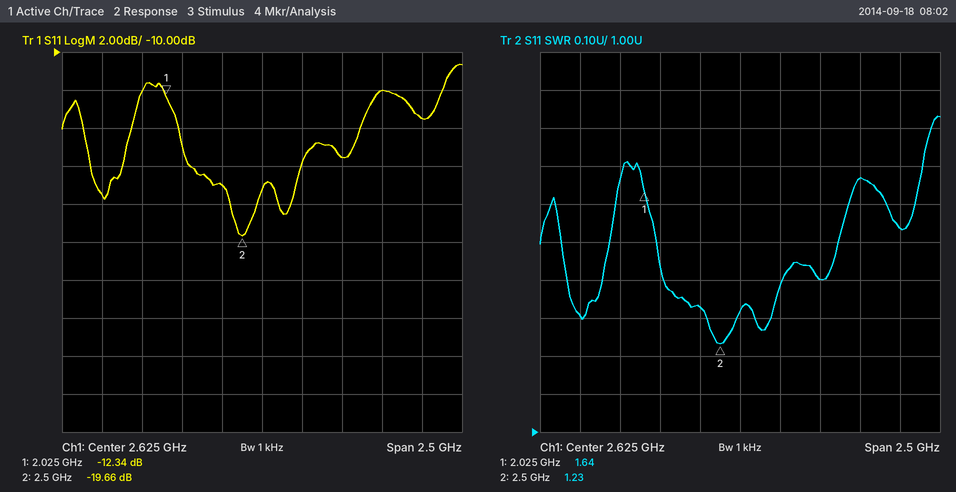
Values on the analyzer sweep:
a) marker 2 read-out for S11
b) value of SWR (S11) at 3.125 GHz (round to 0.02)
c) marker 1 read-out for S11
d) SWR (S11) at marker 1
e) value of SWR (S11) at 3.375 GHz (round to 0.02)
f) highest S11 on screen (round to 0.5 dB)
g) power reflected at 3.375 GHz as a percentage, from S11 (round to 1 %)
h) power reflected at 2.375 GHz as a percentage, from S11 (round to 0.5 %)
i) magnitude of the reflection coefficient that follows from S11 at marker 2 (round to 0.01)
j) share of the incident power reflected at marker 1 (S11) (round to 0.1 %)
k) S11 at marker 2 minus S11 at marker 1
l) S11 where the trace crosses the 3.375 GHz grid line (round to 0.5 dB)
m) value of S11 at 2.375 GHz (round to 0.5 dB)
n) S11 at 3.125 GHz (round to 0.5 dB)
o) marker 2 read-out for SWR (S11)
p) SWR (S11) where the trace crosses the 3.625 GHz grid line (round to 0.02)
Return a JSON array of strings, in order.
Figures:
["-19.66 dB", "1.40", "-12.34 dB", "1.64", "1.66", "-10.5 dB", "6 %", "2.0 %", "0.10", "5.8 %", "-7.32 dB", "-12.0 dB", "-17.0 dB", "-15.5 dB", "1.23", "1.54"]
